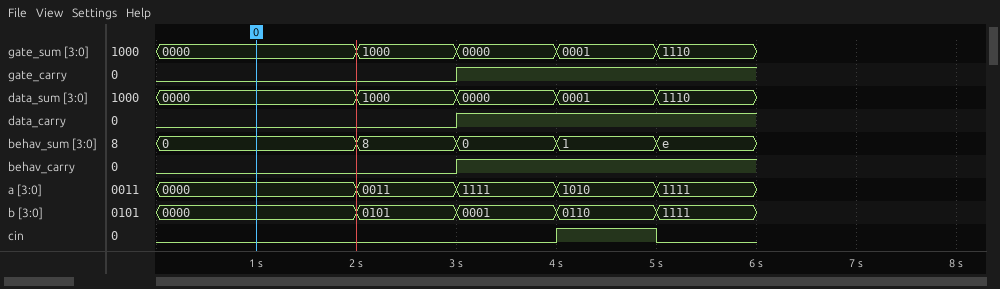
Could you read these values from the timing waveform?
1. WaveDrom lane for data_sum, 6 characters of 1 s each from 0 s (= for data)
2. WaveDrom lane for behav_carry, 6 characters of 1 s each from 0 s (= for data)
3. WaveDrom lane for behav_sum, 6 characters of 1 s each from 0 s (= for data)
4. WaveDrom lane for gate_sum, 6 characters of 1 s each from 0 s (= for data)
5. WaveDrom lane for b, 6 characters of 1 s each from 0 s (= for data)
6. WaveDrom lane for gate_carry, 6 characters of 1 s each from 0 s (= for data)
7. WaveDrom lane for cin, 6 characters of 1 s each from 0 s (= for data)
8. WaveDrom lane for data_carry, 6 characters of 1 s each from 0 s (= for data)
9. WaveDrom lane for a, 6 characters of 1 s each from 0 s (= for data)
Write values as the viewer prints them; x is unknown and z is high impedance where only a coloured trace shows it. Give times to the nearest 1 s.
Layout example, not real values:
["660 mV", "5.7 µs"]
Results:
["{name: 'data_sum', wave: '=.====', data: '0000 1000 0000 0001 1110'}", "{name: 'behav_carry', wave: '0..1..'}", "{name: 'behav_sum', wave: '=.====', data: '0 8 0 1 e'}", "{name: 'gate_sum', wave: '=.====', data: '0000 1000 0000 0001 1110'}", "{name: 'b', wave: '=.====', data: '0000 0101 0001 0110 1111'}", "{name: 'gate_carry', wave: '0..1..'}", "{name: 'cin', wave: '0...10'}", "{name: 'data_carry', wave: '0..1..'}", "{name: 'a', wave: '=.====', data: '0000 0011 1111 1010 1111'}"]
